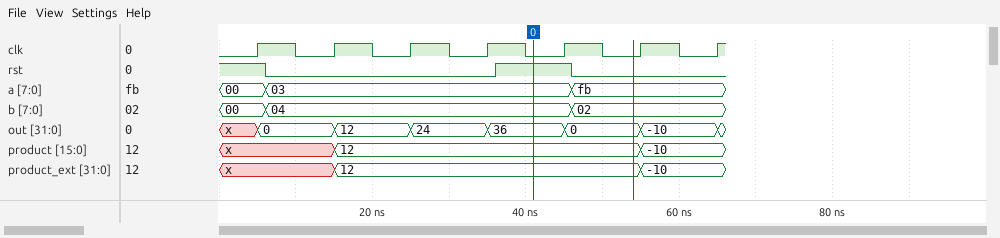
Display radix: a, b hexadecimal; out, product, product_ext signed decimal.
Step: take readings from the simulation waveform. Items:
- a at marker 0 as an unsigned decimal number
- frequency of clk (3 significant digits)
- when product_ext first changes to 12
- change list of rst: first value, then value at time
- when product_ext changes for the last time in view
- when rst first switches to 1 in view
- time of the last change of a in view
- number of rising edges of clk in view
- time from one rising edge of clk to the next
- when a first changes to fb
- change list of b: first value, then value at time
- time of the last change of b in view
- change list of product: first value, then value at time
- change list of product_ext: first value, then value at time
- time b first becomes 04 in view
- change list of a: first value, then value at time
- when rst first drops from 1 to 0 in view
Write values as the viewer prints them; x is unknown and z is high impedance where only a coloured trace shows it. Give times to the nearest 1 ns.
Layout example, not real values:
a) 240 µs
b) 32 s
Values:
a) 3
b) 100 MHz
c) 15 ns
d) 1, 0 at 6 ns, 1 at 36 ns, 0 at 46 ns
e) 55 ns
f) 36 ns
g) 46 ns
h) 7
i) 10 ns
j) 46 ns
k) 00, 04 at 6 ns, 02 at 46 ns
l) 46 ns
m) x, 12 at 15 ns, -10 at 55 ns
n) x, 12 at 15 ns, -10 at 55 ns
o) 6 ns
p) 00, 03 at 6 ns, fb at 46 ns
q) 6 ns
